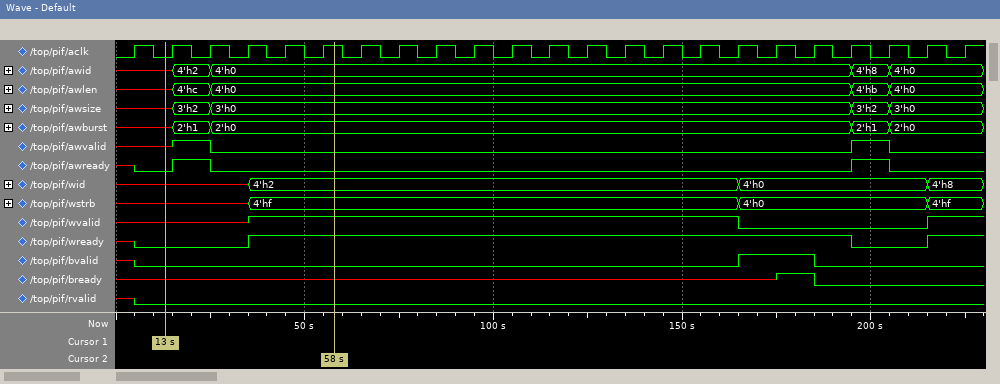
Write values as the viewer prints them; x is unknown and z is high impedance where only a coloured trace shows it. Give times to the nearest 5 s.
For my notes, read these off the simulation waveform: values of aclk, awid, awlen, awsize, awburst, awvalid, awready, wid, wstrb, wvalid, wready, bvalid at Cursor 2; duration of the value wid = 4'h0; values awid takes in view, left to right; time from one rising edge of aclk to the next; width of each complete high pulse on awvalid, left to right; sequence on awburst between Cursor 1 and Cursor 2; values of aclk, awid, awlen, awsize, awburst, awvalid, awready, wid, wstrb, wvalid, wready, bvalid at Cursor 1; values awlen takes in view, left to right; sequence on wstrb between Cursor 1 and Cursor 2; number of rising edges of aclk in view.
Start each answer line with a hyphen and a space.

- aclk=1, awid=4'h0, awlen=4'h0, awsize=3'h0, awburst=2'h0, awvalid=0, awready=0, wid=4'h2, wstrb=4'hf, wvalid=1, wready=1, bvalid=0
- 50 s
- x, 4'h2, 4'h0, 4'h8, 4'h0
- 10 s
- 10 s
- x, 2'h1, 2'h0
- aclk=0, awid=x, awlen=x, awsize=x, awburst=x, awvalid=x, awready=0, wid=x, wstrb=x, wvalid=x, wready=0, bvalid=0
- x, 4'hc, 4'h0, 4'hb, 4'h0
- x, 4'hf
- 23
